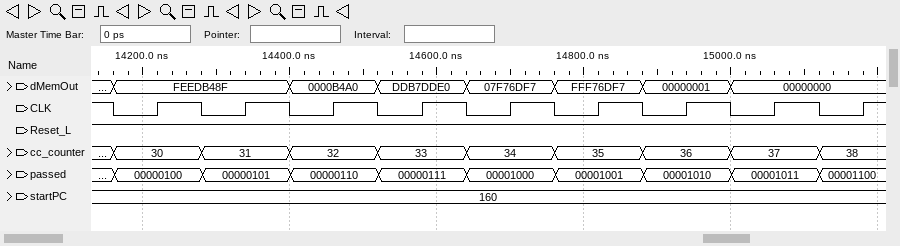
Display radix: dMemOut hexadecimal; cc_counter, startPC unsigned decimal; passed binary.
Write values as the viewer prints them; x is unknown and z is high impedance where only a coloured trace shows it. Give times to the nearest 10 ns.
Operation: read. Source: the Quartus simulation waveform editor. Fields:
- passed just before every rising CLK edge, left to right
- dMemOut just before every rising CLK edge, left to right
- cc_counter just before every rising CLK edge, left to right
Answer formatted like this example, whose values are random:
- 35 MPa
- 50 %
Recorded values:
- 00000100, 00000101, 00000110, 00000111, 00001000, 00001001, 00001010, 00001011, 00001100
- FEEDB48F, FEEDB48F, 0000B4A0, DDB7DDE0, 07F76DF7, FFF76DF7, 00000001, 00000000, 00000000
- 30, 31, 32, 33, 34, 35, 36, 37, 38
